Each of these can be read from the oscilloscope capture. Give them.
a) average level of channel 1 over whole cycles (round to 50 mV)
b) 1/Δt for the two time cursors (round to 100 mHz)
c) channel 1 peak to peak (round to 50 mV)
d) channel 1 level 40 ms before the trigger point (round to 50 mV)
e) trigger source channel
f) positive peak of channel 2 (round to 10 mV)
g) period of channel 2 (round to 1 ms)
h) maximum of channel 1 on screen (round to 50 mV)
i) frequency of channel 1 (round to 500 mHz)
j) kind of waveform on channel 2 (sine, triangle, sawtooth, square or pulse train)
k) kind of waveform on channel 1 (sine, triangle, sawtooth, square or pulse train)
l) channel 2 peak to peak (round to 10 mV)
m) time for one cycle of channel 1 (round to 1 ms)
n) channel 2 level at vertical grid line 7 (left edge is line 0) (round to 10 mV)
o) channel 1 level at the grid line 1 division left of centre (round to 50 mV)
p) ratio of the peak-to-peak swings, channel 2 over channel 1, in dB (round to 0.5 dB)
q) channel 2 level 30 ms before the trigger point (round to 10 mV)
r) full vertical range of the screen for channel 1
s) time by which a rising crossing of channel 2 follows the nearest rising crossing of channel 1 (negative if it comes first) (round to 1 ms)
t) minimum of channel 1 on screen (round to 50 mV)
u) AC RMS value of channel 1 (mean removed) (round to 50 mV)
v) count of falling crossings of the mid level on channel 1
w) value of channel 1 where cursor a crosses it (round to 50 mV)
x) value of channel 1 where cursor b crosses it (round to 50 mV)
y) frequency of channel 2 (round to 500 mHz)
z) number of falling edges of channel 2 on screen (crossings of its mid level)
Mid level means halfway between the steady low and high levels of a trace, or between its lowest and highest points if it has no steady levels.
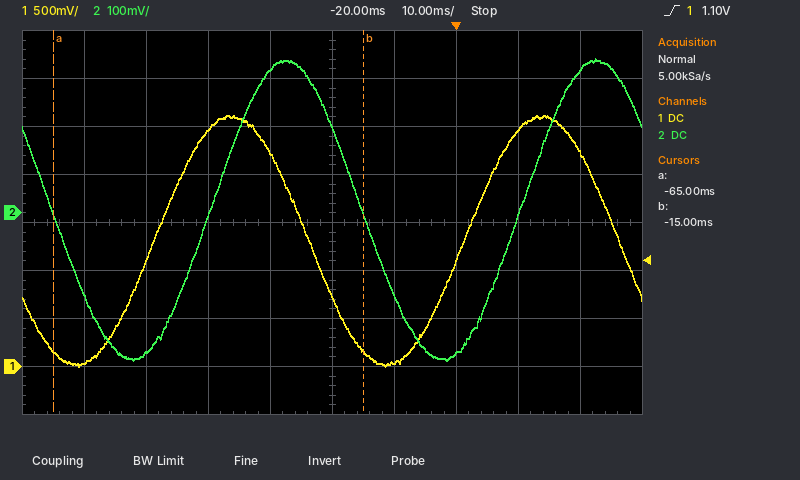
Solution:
1.30 V
20.0 Hz
2.60 V
2.45 V
channel 1
320 mV
50 ms
2.60 V
20.0 Hz
sine
sine
630 mV
50 ms
-290 mV
2.25 V
-12.5 dB
300 mV
4 V
+9 ms
0 mV
900 mV
2
150 mV
150 mV
20.0 Hz
2
